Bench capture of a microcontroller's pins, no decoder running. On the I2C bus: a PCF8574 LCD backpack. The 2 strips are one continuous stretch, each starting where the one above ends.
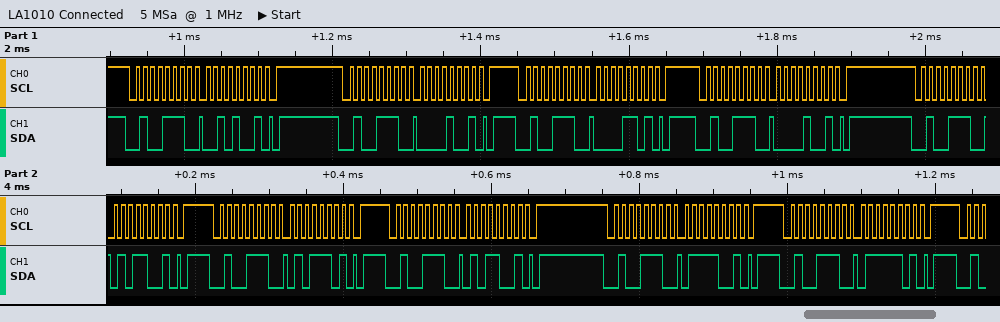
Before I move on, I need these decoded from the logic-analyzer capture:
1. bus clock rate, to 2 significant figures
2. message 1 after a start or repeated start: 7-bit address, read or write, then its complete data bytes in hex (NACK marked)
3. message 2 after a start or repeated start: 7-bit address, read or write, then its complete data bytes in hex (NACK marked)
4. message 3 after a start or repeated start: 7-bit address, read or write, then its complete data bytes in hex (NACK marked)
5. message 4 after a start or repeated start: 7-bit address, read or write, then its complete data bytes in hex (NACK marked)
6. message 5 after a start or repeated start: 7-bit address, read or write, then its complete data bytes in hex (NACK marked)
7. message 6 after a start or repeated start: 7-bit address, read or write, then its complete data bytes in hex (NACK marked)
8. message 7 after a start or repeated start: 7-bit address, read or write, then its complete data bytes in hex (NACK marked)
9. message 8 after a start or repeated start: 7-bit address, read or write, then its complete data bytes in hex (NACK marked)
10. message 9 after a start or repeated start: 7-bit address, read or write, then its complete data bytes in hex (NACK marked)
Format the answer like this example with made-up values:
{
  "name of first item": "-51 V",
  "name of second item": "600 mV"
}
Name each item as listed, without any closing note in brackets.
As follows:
{
  "bus clock rate, to 2 significant figures": "100 kHz",
  "message 1 after a start or repeated start: 7-bit address, read or write, then its complete data bytes in hex": "0x27 write: 29",
  "message 2 after a start or repeated start: 7-bit address, read or write, then its complete data bytes in hex": "0x27 write: 09",
  "message 3 after a start or repeated start: 7-bit address, read or write, then its complete data bytes in hex": "0x27 write: 0D",
  "message 4 after a start or repeated start: 7-bit address, read or write, then its complete data bytes in hex": "0x27 write: 09",
  "message 5 after a start or repeated start: 7-bit address, read or write, then its complete data bytes in hex": "0x27 write: 59",
  "message 6 after a start or repeated start: 7-bit address, read or write, then its complete data bytes in hex": "0x27 write: 5D",
  "message 7 after a start or repeated start: 7-bit address, read or write, then its complete data bytes in hex": "0x27 write: 59",
  "message 8 after a start or repeated start: 7-bit address, read or write, then its complete data bytes in hex": "0x27 write: 79",
  "message 9 after a start or repeated start: 7-bit address, read or write, then its complete data bytes in hex": "0x27 write: 7D"
}
